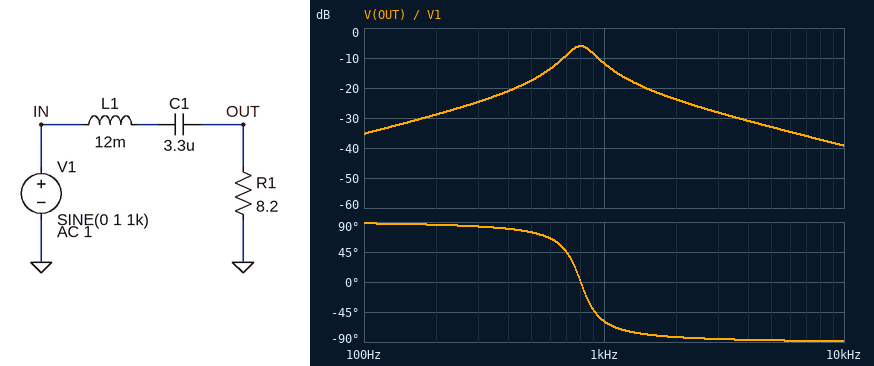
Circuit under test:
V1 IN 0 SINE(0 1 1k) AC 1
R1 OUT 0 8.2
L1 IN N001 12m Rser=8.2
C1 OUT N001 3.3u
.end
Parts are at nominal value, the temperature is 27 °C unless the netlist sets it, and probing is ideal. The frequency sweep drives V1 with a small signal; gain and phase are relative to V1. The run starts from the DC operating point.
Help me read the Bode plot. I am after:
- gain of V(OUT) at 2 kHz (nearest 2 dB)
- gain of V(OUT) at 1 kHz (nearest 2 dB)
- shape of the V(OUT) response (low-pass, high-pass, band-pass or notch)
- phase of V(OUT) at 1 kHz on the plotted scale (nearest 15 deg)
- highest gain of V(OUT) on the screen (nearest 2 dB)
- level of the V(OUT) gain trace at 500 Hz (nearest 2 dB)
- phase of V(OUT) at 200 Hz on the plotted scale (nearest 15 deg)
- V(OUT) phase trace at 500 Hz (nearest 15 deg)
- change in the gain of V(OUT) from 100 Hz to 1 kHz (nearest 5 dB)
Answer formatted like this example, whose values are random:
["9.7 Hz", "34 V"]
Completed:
["-24 dB", "-12 dB", "band-pass", "-60 deg", "-6 dB", "-18 dB", "90 deg", "75 deg", "25 dB"]
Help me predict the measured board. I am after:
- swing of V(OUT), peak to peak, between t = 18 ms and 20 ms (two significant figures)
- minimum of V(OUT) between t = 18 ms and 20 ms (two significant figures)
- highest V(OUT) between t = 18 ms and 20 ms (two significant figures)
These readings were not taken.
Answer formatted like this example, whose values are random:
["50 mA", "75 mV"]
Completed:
["520 mV", "-260 mV", "260 mV"]
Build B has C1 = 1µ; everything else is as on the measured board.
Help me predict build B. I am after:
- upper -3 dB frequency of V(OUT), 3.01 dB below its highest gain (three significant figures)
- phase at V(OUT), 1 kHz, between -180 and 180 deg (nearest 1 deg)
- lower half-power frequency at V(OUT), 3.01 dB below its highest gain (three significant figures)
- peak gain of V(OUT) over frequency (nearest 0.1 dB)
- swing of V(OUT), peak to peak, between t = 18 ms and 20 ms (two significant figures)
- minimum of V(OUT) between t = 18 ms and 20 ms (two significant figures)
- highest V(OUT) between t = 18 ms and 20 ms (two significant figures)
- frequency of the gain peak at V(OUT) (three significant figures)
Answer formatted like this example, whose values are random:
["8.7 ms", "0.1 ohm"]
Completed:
["1.57 kHz", "79 deg", "1.35 kHz", "-6.0 dB", "190 mV", "-96 mV", "96 mV", "1.45 kHz"]
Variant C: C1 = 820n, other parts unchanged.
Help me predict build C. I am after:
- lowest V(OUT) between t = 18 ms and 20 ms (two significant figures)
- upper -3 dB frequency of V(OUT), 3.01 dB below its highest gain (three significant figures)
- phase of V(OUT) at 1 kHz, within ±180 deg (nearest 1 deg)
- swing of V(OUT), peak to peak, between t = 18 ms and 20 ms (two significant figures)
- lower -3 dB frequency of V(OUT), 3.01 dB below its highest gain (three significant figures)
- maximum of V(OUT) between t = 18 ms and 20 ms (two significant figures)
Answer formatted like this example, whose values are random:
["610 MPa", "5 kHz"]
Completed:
["-68 mV", "1.72 kHz", "82 deg", "140 mV", "1.50 kHz", "68 mV"]
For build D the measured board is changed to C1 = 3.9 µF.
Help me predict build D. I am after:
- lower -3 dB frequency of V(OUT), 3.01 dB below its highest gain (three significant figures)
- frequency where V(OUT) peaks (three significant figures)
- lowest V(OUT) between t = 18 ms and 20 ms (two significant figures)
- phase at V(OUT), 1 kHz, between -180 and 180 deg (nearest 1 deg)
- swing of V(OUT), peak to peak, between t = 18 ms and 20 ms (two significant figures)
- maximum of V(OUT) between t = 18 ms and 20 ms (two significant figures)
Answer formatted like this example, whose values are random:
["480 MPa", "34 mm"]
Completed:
["635 Hz", "736 Hz", "-210 mV", "-65 deg", "430 mV", "210 mV"]
